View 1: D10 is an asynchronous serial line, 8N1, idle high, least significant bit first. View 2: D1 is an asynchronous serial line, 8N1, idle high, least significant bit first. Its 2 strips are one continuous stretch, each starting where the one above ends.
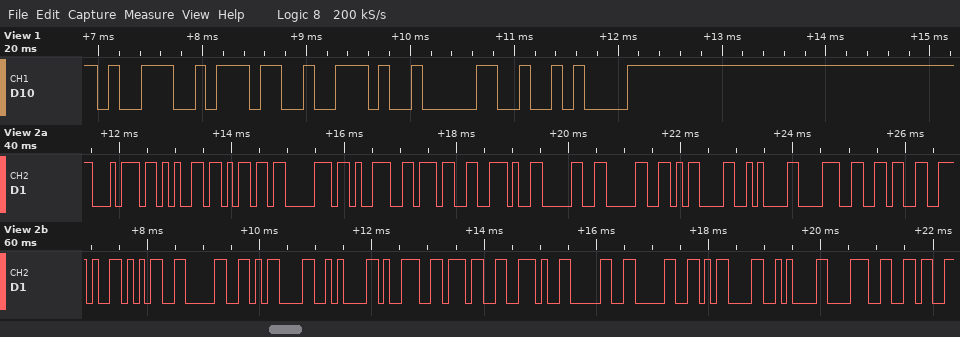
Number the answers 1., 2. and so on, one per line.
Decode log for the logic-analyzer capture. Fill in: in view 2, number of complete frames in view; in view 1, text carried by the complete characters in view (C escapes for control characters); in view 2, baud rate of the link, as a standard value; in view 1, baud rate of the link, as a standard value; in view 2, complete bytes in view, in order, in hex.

1. 27
2. "97.0\n"
3. 9600 baud
4. 9600 baud
5. 74 65 6D 70 39 37 2E 30 30 0D 0A 38 36 2E 35 30 0D 0A 39 37 2E 30 30 0D 0A 38 36
